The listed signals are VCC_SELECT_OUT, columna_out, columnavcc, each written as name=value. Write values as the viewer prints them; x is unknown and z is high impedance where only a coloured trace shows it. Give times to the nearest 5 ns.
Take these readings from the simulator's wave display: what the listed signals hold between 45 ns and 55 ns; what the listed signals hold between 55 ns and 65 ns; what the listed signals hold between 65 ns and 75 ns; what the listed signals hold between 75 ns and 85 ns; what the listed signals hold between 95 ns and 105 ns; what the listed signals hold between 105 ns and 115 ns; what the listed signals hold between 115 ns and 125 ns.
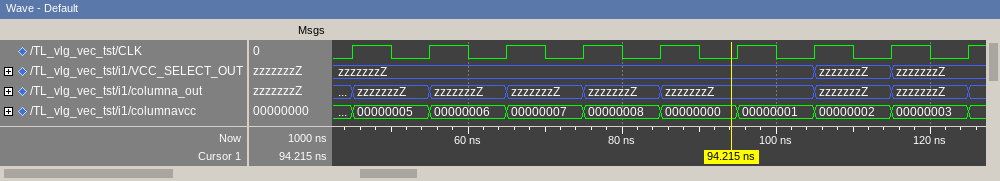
VCC_SELECT_OUT=zzzzzzzZ, columna_out=zzzzzzzZ, columnavcc=00000005
VCC_SELECT_OUT=zzzzzzzZ, columna_out=zzzzzzzZ, columnavcc=00000006
VCC_SELECT_OUT=zzzzzzzZ, columna_out=zzzzzzzZ, columnavcc=00000007
VCC_SELECT_OUT=zzzzzzzZ, columna_out=zzzzzzzZ, columnavcc=00000008
VCC_SELECT_OUT=zzzzzzzZ, columna_out=zzzzzzzZ, columnavcc=00000001
VCC_SELECT_OUT=zzzzzzzZ, columna_out=zzzzzzzZ, columnavcc=00000002
VCC_SELECT_OUT=zzzzzzzZ, columna_out=zzzzzzzZ, columnavcc=00000003
